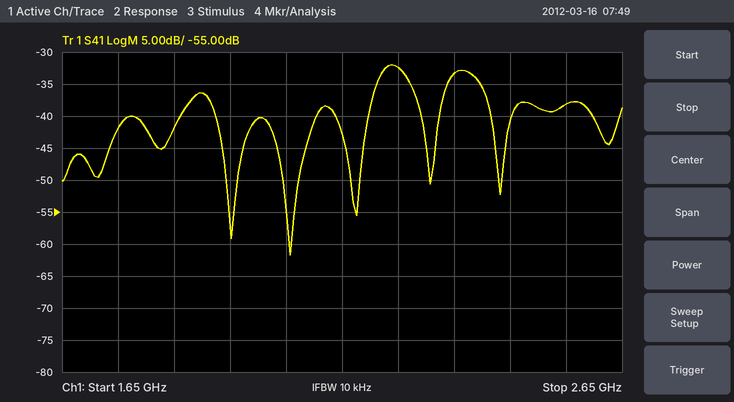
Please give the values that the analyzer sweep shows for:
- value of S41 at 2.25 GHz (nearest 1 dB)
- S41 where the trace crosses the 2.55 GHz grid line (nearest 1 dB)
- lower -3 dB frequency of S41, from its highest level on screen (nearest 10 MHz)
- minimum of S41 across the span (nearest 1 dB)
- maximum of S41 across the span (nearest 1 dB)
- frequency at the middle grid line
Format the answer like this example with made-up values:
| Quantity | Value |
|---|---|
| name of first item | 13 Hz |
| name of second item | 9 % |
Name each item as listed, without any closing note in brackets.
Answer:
| Quantity | Value |
|---|---|
| value of S41 at 2.25 GHz | -32 dB |
| S41 where the trace crosses the 2.55 GHz grid line | -38 dB |
| lower -3 dB frequency of S41, from its highest level on screen | 2.21 GHz |
| minimum of S41 across the span | -62 dB |
| maximum of S41 across the span | -32 dB |
| frequency at the middle grid line | 2.15 GHz |
